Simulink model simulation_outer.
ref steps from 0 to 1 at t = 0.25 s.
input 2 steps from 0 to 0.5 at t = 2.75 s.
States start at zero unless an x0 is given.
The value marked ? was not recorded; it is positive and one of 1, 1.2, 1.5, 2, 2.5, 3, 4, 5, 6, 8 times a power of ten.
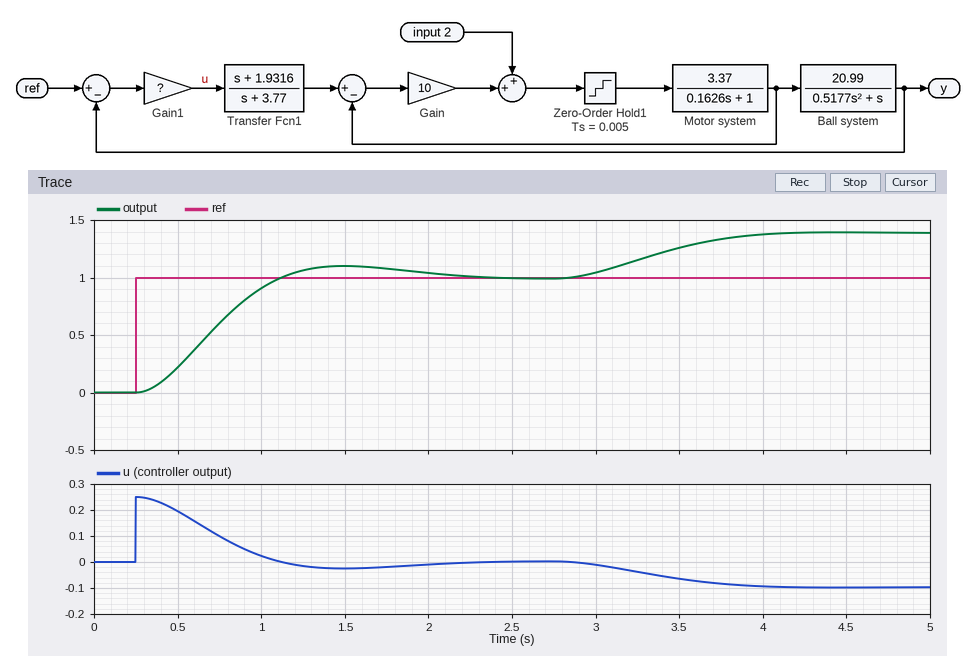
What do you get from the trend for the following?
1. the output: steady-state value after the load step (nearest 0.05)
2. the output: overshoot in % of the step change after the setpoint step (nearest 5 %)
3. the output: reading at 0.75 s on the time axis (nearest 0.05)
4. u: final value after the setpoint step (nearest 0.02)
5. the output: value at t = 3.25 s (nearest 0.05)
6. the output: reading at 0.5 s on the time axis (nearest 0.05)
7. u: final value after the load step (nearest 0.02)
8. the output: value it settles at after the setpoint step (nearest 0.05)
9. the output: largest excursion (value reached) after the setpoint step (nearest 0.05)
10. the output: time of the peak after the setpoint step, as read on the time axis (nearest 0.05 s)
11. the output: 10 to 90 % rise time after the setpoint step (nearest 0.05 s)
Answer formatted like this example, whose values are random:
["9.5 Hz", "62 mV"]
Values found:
["1.40", "10 %", "0.60", "0.00", "1.15", "0.20", "-0.10", "1.00", "1.10", "1.50 s", "0.60 s"]
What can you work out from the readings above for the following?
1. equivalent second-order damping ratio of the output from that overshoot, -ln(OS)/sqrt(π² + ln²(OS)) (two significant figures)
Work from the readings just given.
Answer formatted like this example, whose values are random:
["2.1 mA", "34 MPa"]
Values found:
["0.59"]
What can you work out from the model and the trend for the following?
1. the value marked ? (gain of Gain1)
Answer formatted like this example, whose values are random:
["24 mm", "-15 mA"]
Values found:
["0.25"]
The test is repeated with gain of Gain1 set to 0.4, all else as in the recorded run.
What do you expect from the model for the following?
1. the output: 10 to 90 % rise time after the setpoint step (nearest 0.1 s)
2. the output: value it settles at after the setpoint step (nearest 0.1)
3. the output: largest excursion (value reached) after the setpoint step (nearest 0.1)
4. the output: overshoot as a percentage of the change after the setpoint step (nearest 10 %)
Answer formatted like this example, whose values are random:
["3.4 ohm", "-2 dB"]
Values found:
["0.4 s", "1.0", "1.2", "20 %"]
